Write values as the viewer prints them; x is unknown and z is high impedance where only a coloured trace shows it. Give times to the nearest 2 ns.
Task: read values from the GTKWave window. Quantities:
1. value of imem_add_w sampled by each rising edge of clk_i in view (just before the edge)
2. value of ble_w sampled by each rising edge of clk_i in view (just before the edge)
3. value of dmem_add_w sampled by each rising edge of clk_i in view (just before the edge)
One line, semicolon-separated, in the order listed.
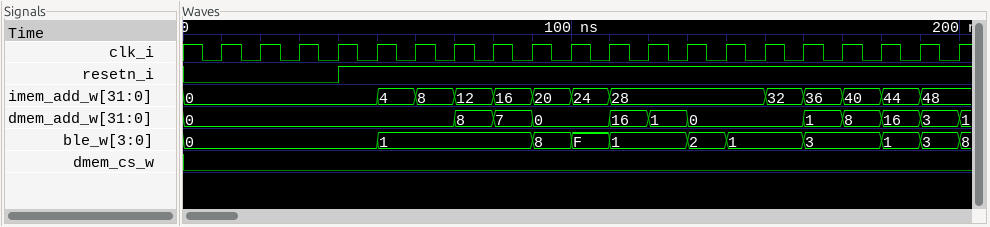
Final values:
0, 0, 0, 0, 0, 4, 8, 12, 16, 20, 24, 28, 28, 28, 28, 32, 36, 40, 44, 48; 0, 0, 0, 0, 0, 1, 1, 1, 1, 8, F, 1, 1, 2, 1, 1, 3, 3, 1, 3; 0, 0, 0, 0, 0, 0, 0, 8, 7, 0, 0, 16, 1, 0, 0, 0, 1, 8, 16, 3
